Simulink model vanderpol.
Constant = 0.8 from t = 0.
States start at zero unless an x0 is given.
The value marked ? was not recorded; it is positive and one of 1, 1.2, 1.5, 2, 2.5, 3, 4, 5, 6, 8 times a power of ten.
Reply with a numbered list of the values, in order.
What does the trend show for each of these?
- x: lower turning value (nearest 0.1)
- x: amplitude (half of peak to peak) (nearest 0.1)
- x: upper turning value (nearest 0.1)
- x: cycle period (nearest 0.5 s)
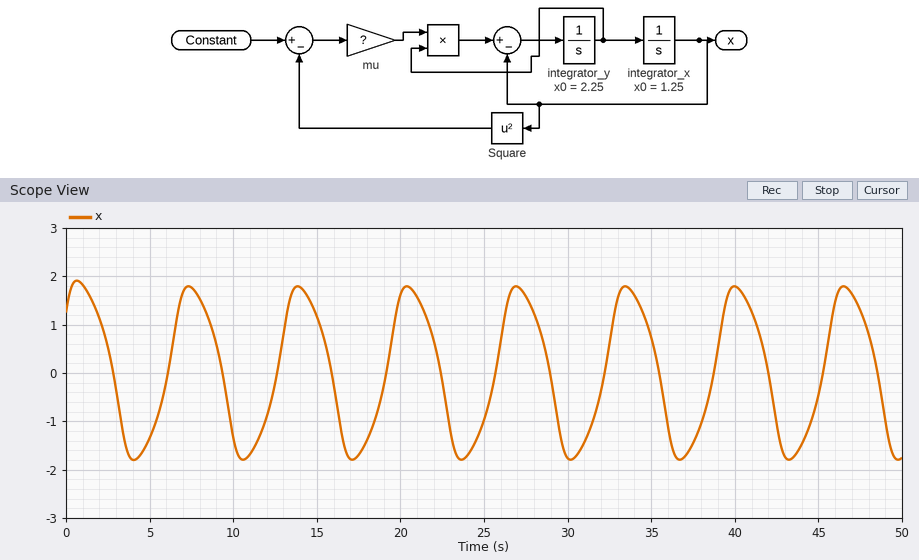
1. -1.8
2. 1.8
3. 1.8
4. 6.5 s
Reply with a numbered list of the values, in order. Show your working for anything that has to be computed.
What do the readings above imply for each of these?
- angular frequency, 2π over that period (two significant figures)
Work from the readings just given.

1. 2π / 6.5 = 0.97 rad/s
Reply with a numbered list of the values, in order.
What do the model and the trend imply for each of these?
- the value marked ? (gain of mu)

1. 1
